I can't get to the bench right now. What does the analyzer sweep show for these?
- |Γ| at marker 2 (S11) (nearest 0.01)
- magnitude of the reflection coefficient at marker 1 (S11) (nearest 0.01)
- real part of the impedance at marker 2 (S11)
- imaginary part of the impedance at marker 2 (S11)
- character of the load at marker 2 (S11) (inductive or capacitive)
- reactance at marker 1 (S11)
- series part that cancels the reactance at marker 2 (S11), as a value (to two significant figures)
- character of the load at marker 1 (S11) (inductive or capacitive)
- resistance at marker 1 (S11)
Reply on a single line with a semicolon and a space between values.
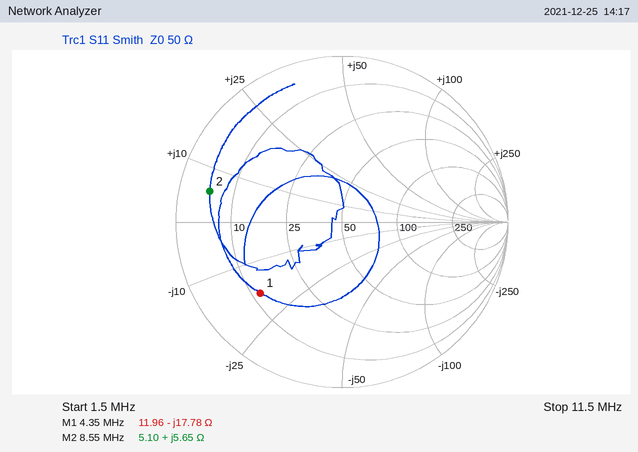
0.82; 0.65; 5.10 Ω; +5.65 Ω; inductive; -17.78 Ω; 3.3 nF; capacitive; 11.96 Ω
